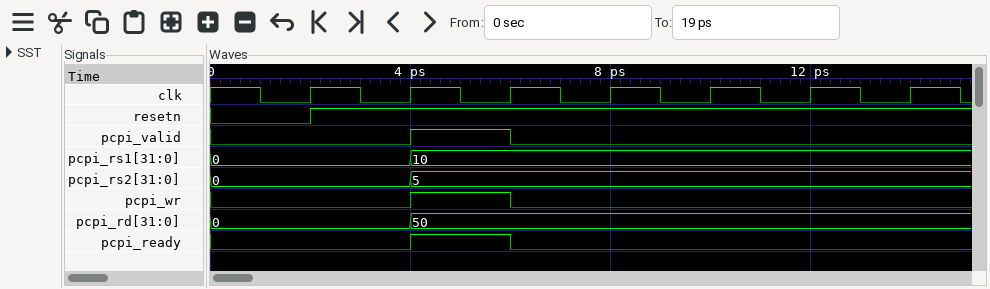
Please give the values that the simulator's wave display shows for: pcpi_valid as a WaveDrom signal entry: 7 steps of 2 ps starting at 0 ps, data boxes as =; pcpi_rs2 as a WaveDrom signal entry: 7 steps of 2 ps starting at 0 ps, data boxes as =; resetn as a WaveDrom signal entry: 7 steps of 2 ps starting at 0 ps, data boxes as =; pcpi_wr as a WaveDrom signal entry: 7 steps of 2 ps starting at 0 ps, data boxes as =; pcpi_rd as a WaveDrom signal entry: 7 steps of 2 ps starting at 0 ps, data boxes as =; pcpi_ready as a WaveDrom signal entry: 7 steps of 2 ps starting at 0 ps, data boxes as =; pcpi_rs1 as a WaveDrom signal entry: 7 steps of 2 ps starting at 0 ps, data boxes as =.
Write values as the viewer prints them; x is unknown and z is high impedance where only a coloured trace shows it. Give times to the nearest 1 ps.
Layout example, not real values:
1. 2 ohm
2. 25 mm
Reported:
1. {name: 'pcpi_valid', wave: '0.10...'}
2. {name: 'pcpi_rs2', wave: '=.=....', data: '0 5'}
3. {name: 'resetn', wave: '01.....'}
4. {name: 'pcpi_wr', wave: '0.10...'}
5. {name: 'pcpi_rd', wave: '=.=....', data: '0 50'}
6. {name: 'pcpi_ready', wave: '0.10...'}
7. {name: 'pcpi_rs1', wave: '=.=....', data: '0 10'}
